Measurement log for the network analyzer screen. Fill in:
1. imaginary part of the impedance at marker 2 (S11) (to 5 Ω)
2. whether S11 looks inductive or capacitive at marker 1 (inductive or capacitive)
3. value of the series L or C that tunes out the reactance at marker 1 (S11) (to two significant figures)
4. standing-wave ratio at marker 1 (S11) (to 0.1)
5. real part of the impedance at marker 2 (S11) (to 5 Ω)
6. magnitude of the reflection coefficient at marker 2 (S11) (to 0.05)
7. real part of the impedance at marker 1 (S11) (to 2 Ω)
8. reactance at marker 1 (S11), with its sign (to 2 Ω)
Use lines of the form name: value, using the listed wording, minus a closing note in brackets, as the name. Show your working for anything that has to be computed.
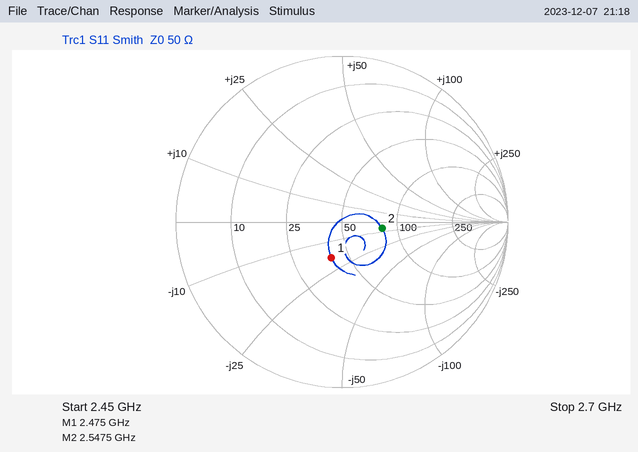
imaginary part of the impedance at marker 2 (S11): -5 Ω
whether S11 looks inductive or capacitive at marker 1: capacitive
value of the series L or C that tunes out the reactance at marker 1 (S11): L = 18 Ω/(2π × 2.475 GHz) ≈ 1.2 nH
standing-wave ratio at marker 1 (S11): 1.6
real part of the impedance at marker 2 (S11): 80 Ω
magnitude of the reflection coefficient at marker 2 (S11): 0.25
real part of the impedance at marker 1 (S11): 40 Ω
reactance at marker 1 (S11), with its sign: -18 Ω
